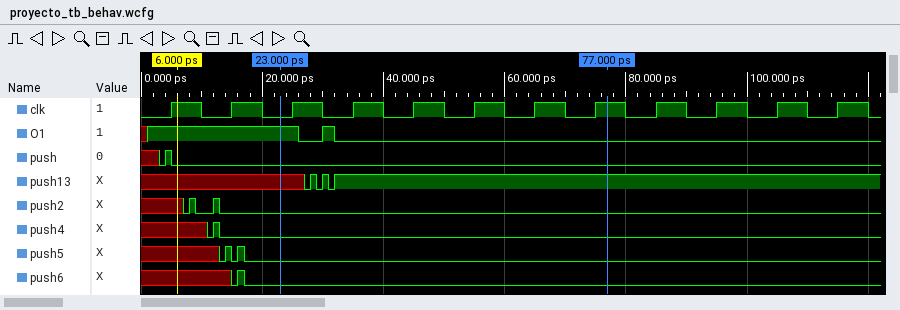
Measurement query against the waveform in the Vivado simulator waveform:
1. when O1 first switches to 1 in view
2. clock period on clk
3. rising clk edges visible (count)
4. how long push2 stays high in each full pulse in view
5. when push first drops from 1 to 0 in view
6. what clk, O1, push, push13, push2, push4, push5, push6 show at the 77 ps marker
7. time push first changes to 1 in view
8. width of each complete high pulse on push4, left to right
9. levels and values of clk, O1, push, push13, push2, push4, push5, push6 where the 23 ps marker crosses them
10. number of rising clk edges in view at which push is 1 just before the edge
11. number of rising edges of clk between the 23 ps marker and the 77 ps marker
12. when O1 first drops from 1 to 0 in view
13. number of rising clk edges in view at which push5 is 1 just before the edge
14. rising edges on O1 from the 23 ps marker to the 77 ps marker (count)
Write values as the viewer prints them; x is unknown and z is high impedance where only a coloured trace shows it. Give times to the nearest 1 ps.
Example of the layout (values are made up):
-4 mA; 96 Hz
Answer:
1 ps; 10 ps; 12; 1 ps, 1 ps; 5 ps; clk=1, O1=0, push=0, push13=1, push2=0, push4=0, push5=0, push6=0; 4 ps; 1 ps; clk=0, O1=1, push=0, push13=x, push2=0, push4=0, push5=0, push6=0; 1; 6; 26 ps; 1; 1
